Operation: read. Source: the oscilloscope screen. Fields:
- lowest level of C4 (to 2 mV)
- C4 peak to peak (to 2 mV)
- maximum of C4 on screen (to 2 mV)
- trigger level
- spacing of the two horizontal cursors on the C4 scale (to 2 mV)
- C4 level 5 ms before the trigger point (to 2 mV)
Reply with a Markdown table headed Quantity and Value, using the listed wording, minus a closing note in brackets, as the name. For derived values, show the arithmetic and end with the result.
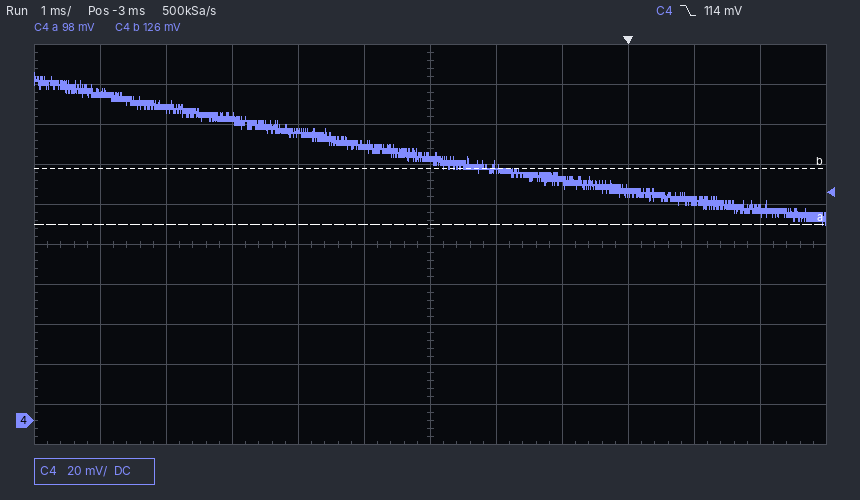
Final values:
| Quantity | Value |
|---|---|
| lowest level of C4 | 98 mV |
| C4 peak to peak | 174 mV − (98 mV) = 76 mV |
| maximum of C4 on screen | 174 mV |
| trigger level | 114 mV |
| spacing of the two horizontal cursors on the C4 scale | 28 mV |
| C4 level 5 ms before the trigger point | 144 mV |
